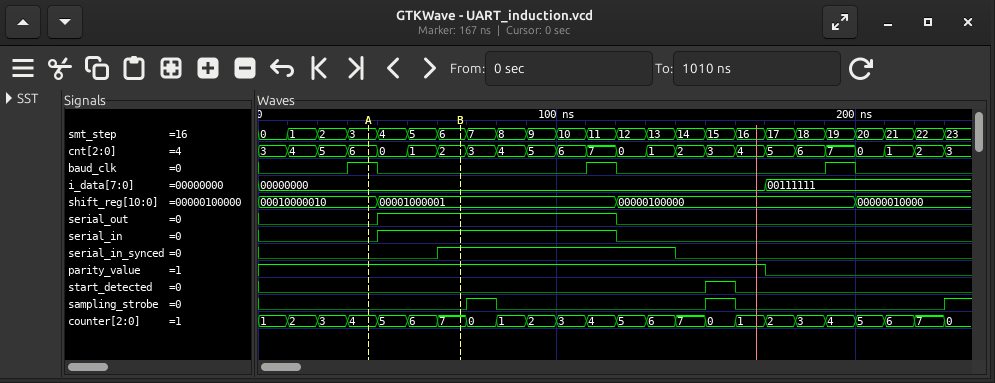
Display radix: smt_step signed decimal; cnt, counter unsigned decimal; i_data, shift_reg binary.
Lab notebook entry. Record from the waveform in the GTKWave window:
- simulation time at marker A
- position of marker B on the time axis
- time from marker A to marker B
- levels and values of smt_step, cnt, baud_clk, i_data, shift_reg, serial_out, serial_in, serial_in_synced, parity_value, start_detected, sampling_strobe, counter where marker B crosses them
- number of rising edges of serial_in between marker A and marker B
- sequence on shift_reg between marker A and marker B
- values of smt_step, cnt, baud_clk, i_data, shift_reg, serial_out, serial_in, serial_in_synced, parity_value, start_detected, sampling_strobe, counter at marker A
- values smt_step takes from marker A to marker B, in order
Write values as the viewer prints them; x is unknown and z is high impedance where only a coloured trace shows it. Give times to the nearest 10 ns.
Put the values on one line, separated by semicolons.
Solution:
40 ns; 70 ns; 30 ns; smt_step=6, cnt=2, baud_clk=0, i_data=00000000, shift_reg=00001000001, serial_out=1, serial_in=1, serial_in_synced=1, parity_value=1, start_detected=0, sampling_strobe=0, counter=7; 1; 00010000010, 00001000001; smt_step=3, cnt=6, baud_clk=1, i_data=00000000, shift_reg=00010000010, serial_out=0, serial_in=0, serial_in_synced=0, parity_value=1, start_detected=0, sampling_strobe=0, counter=4; 3, 4, 5, 6
